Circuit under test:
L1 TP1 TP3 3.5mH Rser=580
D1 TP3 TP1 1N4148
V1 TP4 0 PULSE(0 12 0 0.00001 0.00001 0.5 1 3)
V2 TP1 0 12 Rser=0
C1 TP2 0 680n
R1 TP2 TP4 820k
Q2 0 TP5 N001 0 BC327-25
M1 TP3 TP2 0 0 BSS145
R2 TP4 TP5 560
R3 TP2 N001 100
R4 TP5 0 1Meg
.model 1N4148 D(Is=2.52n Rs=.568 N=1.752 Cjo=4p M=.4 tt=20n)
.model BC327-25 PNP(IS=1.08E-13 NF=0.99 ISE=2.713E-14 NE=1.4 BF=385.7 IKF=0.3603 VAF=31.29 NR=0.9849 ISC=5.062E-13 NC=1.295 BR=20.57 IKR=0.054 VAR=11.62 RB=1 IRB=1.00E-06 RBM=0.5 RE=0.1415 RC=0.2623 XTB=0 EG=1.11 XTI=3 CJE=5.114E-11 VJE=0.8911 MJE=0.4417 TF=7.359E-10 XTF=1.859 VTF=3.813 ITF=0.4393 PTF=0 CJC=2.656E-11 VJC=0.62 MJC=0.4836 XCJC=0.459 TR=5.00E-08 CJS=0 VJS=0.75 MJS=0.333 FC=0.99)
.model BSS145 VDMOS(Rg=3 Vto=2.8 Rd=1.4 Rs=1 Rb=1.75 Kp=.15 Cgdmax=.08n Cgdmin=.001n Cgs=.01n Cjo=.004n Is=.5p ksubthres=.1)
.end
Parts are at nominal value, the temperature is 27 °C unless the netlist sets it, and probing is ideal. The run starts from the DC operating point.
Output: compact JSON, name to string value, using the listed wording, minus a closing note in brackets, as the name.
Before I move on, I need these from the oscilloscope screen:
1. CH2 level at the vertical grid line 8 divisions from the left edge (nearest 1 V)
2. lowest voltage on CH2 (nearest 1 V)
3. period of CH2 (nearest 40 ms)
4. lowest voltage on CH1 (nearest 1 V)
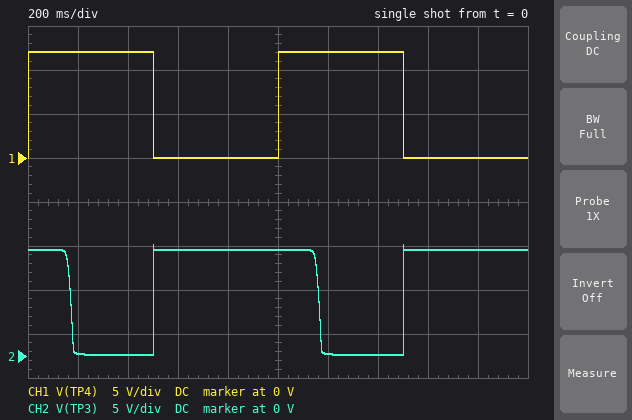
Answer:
{"CH2 level at the vertical grid line 8 divisions from the left edge": "12 V", "lowest voltage on CH2": "0 V", "period of CH2": "1.00 s", "lowest voltage on CH1": "0 V"}
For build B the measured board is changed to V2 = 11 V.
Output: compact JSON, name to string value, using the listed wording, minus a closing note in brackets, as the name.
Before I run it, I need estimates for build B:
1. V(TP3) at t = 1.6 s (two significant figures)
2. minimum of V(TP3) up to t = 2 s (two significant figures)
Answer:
{"V(TP3) at t = 1.6 s": "11 V", "minimum of V(TP3) up to t = 2 s": "74 mV"}
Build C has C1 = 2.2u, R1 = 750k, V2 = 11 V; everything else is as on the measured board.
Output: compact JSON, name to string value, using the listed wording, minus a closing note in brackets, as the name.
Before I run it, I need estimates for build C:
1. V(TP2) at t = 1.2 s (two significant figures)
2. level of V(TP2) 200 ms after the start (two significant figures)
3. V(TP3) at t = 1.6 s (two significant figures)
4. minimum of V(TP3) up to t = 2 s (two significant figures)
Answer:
{"V(TP2) at t = 1.2 s": "1.6 V", "level of V(TP2) 200 ms after the start": "1.4 V", "V(TP3) at t = 1.6 s": "11 V", "minimum of V(TP3) up to t = 2 s": "380 mV"}
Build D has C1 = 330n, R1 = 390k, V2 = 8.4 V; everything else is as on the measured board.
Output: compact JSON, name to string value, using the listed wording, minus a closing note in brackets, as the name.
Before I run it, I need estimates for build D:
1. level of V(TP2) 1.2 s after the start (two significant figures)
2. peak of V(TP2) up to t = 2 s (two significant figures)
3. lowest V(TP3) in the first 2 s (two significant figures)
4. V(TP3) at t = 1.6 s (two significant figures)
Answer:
{"level of V(TP2) 1.2 s after the start": "9.5 V", "peak of V(TP2) up to t = 2 s": "12 V", "lowest V(TP3) in the first 2 s": "45 mV", "V(TP3) at t = 1.6 s": "8.4 V"}
